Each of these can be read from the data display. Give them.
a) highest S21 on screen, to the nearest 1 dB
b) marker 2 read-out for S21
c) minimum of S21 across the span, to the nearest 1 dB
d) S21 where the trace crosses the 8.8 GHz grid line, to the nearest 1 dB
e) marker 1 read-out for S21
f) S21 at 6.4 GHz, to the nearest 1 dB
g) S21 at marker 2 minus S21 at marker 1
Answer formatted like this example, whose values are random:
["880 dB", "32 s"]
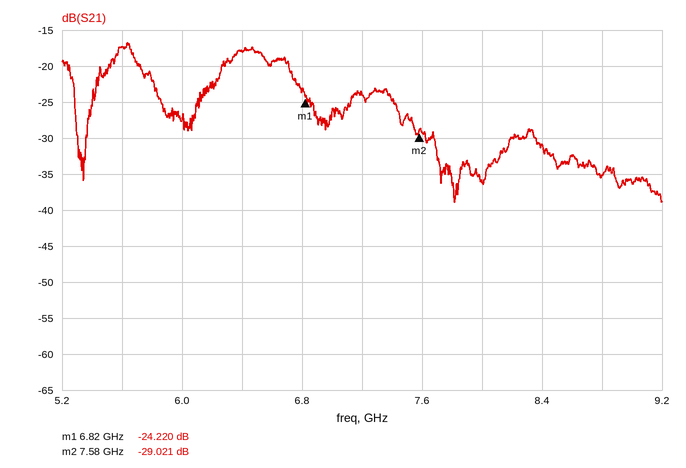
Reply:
["-17 dB", "-29.021 dB", "-39 dB", "-35 dB", "-24.220 dB", "-18 dB", "-4.801 dB"]
